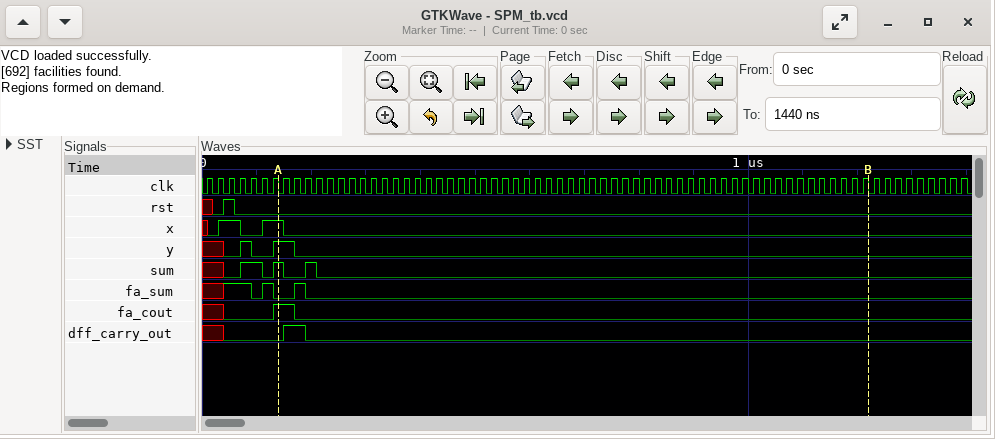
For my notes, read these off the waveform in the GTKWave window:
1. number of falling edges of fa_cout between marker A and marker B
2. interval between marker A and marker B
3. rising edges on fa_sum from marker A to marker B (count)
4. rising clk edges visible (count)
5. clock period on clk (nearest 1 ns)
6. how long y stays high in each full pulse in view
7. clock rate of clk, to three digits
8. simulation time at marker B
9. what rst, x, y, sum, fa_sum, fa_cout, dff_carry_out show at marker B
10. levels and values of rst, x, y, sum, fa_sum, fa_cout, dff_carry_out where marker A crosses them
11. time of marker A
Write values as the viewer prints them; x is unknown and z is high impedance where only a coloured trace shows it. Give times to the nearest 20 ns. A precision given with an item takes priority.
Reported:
1
1080 ns
1
70
20 ns
20 ns, 40 ns
50.0 MHz
1220 ns
rst=0, x=0, y=0, sum=0, fa_sum=0, fa_cout=0, dff_carry_out=0
rst=0, x=1, y=1, sum=1, fa_sum=0, fa_cout=1, dff_carry_out=0
140 ns
